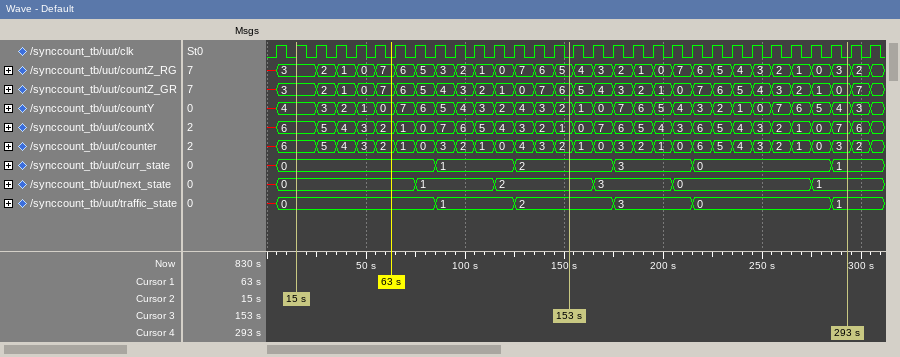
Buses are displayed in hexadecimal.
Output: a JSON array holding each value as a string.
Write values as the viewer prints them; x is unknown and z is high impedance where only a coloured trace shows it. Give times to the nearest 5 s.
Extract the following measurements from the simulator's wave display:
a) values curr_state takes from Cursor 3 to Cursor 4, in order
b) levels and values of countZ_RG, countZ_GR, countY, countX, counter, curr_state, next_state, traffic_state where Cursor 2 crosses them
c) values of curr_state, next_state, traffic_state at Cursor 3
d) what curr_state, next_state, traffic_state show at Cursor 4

["2, 3, 0, 1", "countZ_RG=3, countZ_GR=3, countY=4, countX=6, counter=6, curr_state=0, next_state=0, traffic_state=0", "curr_state=2, next_state=2, traffic_state=2", "curr_state=1, next_state=1, traffic_state=1"]
